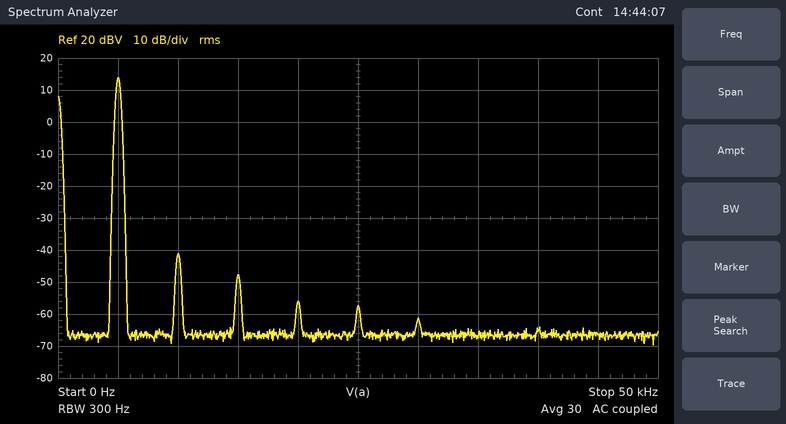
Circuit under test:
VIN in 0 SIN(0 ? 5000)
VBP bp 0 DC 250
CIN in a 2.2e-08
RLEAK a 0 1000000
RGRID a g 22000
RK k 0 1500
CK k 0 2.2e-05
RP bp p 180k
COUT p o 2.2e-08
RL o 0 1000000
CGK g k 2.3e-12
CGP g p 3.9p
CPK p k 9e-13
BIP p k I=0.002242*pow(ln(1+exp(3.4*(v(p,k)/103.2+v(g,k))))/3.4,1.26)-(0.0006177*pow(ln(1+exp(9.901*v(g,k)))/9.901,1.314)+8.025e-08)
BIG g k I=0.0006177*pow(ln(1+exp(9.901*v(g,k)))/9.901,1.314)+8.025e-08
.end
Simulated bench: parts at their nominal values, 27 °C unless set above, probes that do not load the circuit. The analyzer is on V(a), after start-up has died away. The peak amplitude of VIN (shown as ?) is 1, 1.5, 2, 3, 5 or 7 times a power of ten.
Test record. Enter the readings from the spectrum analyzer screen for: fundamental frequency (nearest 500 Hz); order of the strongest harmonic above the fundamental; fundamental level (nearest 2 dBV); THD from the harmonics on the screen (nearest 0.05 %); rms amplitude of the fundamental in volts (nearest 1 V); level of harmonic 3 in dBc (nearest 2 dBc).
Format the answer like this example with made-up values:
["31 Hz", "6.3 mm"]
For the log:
["5.0 kHz", "2", "14 dBV", "0.20 %", "5 V", "-62 dBc"]
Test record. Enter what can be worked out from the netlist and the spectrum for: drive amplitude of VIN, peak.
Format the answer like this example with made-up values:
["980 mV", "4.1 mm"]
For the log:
["7 V"]
